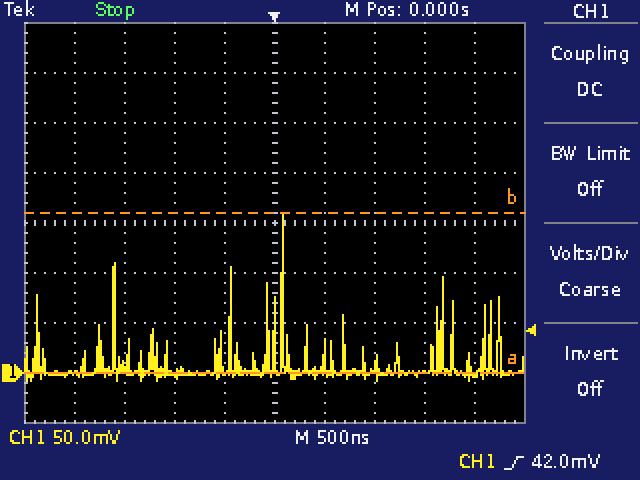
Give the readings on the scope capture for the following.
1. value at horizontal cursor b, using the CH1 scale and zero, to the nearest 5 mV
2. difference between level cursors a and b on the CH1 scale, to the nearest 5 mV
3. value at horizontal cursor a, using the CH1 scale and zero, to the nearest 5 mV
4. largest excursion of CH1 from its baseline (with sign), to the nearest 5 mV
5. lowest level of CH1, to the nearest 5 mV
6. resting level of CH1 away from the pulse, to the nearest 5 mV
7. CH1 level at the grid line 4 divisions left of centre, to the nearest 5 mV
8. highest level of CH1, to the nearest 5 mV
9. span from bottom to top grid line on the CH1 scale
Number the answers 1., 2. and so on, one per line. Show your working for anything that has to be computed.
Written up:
1. 160 mV
2. 160 mV
3. 0 mV
4. 160 mV − (0 mV) = +160 mV
5. -10 mV
6. 0 mV
7. 0 mV
8. 160 mV
9. 400 mV
